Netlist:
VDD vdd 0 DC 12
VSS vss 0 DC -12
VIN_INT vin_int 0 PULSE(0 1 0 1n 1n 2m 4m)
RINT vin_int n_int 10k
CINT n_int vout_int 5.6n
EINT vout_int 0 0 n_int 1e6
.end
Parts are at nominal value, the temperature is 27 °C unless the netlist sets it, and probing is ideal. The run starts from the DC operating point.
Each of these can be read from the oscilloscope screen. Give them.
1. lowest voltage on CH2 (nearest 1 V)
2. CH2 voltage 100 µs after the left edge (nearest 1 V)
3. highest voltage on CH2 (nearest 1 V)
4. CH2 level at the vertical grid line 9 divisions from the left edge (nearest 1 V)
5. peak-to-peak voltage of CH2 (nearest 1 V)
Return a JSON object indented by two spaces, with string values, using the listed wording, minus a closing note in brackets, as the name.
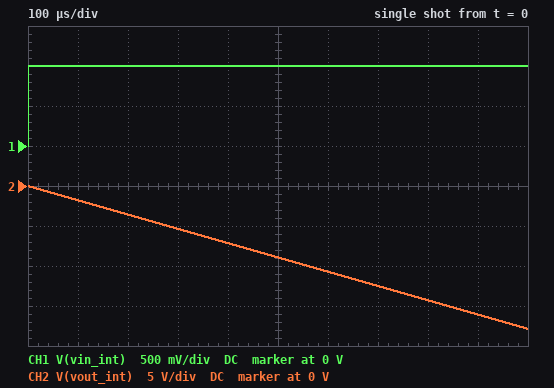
{
  "lowest voltage on CH2": "-18 V",
  "CH2 voltage 100 µs after the left edge": "-2 V",
  "highest voltage on CH2": "0 V",
  "CH2 level at the vertical grid line 9 divisions from the left edge": "-16 V",
  "peak-to-peak voltage of CH2": "18 V"
}
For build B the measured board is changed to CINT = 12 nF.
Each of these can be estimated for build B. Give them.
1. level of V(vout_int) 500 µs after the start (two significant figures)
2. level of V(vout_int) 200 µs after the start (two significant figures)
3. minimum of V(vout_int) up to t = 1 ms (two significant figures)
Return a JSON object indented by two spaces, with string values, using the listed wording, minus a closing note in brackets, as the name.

{
  "level of V(vout_int) 500 µs after the start": "-4.2 V",
  "level of V(vout_int) 200 µs after the start": "-1.7 V",
  "minimum of V(vout_int) up to t = 1 ms": "-8.3 V"
}
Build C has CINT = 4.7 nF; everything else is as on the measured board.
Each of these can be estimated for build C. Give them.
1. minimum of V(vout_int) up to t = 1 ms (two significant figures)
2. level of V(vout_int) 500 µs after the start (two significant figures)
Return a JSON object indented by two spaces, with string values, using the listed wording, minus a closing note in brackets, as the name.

{
  "minimum of V(vout_int) up to t = 1 ms": "-21 V",
  "level of V(vout_int) 500 µs after the start": "-11 V"
}
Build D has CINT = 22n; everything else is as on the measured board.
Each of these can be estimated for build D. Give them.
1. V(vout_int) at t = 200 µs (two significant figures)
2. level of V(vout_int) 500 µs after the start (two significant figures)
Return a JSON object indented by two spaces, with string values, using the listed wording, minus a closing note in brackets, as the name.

{
  "V(vout_int) at t = 200 µs": "-910 mV",
  "level of V(vout_int) 500 µs after the start": "-2.3 V"
}
